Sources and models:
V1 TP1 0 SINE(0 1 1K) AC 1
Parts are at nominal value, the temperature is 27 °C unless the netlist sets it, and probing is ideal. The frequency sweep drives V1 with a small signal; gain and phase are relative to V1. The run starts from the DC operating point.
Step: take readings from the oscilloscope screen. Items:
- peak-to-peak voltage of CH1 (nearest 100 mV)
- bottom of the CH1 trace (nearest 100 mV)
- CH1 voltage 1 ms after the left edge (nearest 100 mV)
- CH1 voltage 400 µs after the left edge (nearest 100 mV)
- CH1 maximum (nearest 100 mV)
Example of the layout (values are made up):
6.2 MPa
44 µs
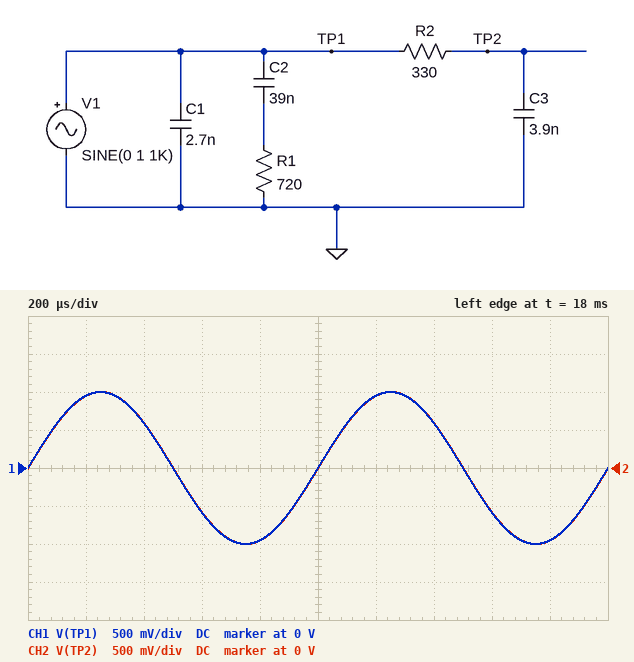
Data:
2.0 V
-1.0 V
0 V
600 mV
1.0 V
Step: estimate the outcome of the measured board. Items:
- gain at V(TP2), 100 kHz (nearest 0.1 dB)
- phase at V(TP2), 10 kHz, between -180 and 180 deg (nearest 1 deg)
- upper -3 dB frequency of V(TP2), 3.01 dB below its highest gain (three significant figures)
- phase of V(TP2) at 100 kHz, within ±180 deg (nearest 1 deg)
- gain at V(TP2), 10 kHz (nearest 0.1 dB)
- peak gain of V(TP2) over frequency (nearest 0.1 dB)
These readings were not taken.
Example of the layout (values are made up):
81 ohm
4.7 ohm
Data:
-2.2 dB
-5 deg
124 kHz
-39 deg
0 dB
0 dB
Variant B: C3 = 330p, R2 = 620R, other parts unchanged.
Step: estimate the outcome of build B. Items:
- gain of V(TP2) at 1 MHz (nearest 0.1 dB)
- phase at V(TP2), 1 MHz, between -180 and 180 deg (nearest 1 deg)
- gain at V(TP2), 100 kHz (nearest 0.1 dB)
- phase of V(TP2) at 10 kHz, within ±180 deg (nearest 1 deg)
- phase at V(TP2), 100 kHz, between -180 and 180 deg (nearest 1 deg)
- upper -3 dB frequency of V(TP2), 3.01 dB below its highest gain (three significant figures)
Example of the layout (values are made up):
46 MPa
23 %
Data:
-4.2 dB
-52 deg
-0.1 dB
-1 deg
-7 deg
778 kHz
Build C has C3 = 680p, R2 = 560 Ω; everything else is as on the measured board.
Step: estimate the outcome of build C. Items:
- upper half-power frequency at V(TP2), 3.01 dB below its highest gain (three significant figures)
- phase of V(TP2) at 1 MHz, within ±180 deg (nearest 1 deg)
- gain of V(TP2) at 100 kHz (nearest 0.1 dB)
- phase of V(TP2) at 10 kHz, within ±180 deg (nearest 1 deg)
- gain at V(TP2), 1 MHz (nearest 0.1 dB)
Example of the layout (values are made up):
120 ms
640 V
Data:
418 kHz
-67 deg
-0.2 dB
-1 deg
-8.3 dB
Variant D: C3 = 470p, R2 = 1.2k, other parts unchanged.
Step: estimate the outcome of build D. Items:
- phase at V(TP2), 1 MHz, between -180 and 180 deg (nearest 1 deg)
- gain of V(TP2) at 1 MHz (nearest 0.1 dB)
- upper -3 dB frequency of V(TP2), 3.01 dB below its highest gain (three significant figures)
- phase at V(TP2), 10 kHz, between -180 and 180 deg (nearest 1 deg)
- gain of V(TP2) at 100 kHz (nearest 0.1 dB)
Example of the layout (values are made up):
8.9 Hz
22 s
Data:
-74 deg
-11.3 dB
282 kHz
-2 deg
-0.5 dB
